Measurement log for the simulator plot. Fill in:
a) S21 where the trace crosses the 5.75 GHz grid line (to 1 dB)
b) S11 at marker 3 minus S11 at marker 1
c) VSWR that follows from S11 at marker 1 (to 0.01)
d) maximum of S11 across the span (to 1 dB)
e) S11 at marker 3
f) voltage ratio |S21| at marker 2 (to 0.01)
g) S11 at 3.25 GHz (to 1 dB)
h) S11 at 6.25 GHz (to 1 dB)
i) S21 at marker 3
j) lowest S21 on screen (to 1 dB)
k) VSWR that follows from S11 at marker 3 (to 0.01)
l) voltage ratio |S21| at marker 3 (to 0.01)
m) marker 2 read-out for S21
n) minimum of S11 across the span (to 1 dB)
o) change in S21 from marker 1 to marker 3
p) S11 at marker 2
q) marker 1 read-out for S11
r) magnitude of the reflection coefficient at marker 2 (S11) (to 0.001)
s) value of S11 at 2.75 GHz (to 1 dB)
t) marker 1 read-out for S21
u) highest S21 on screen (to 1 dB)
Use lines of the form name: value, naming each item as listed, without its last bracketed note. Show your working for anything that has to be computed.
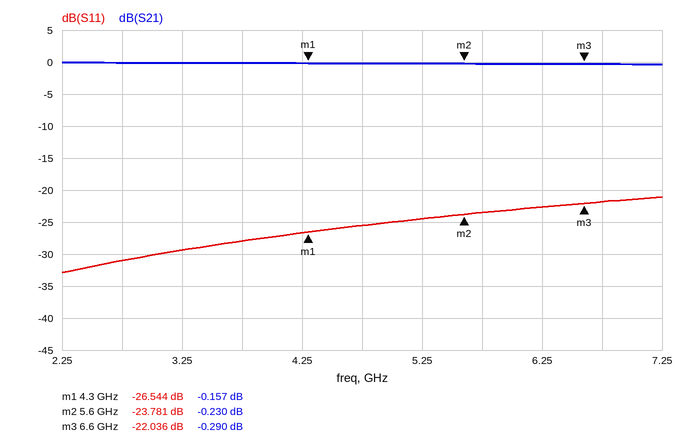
S21 where the trace crosses the 5.75 GHz grid line: 0 dB
S11 at marker 3 minus S11 at marker 1: -22.036 − (-26.544) = 4.508 dB
VSWR that follows from S11 at marker 1: (1 + 0.0471)/(1 − 0.0471) ≈ 1.10
maximum of S11 across the span: -21 dB
S11 at marker 3: -22.036 dB
voltage ratio |S21| at marker 2: 10^(-0.23/20) ≈ 0.97
S11 at 3.25 GHz: -29 dB
S11 at 6.25 GHz: -23 dB
S21 at marker 3: -0.290 dB
lowest S21 on screen: 0 dB
VSWR that follows from S11 at marker 3: (1 + 0.0791)/(1 − 0.0791) ≈ 1.17
voltage ratio |S21| at marker 3: 10^(-0.29/20) ≈ 0.97
marker 2 read-out for S21: -0.230 dB
minimum of S11 across the span: -33 dB
change in S21 from marker 1 to marker 3: -0.29 − (-0.157) = -0.133 dB
S11 at marker 2: -23.781 dB
marker 1 read-out for S11: -26.544 dB
magnitude of the reflection coefficient at marker 2 (S11): 10^(-23.781/20) ≈ 0.065
value of S11 at 2.75 GHz: -31 dB
marker 1 read-out for S21: -0.157 dB
highest S21 on screen: 0 dB
